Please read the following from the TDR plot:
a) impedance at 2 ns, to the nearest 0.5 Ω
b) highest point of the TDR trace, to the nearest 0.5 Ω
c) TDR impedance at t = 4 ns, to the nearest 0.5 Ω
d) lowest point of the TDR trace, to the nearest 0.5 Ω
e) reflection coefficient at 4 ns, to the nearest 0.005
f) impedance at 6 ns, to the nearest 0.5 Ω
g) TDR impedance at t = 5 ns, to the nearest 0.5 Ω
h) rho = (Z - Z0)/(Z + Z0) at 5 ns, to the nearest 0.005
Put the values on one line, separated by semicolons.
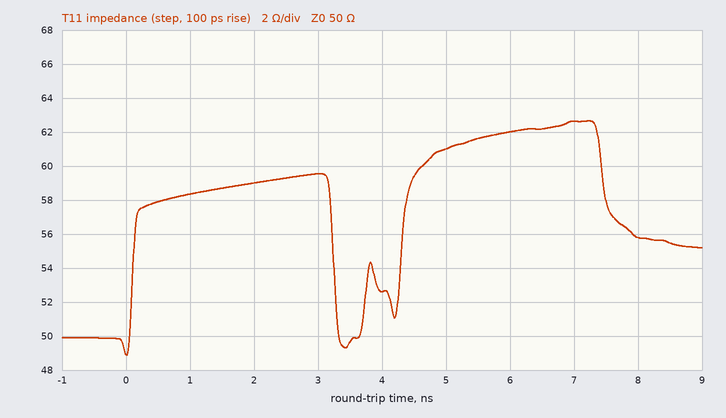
59.0 Ω; 62.5 Ω; 52.5 Ω; 49.0 Ω; +0.025; 62.0 Ω; 61.0 Ω; +0.100
